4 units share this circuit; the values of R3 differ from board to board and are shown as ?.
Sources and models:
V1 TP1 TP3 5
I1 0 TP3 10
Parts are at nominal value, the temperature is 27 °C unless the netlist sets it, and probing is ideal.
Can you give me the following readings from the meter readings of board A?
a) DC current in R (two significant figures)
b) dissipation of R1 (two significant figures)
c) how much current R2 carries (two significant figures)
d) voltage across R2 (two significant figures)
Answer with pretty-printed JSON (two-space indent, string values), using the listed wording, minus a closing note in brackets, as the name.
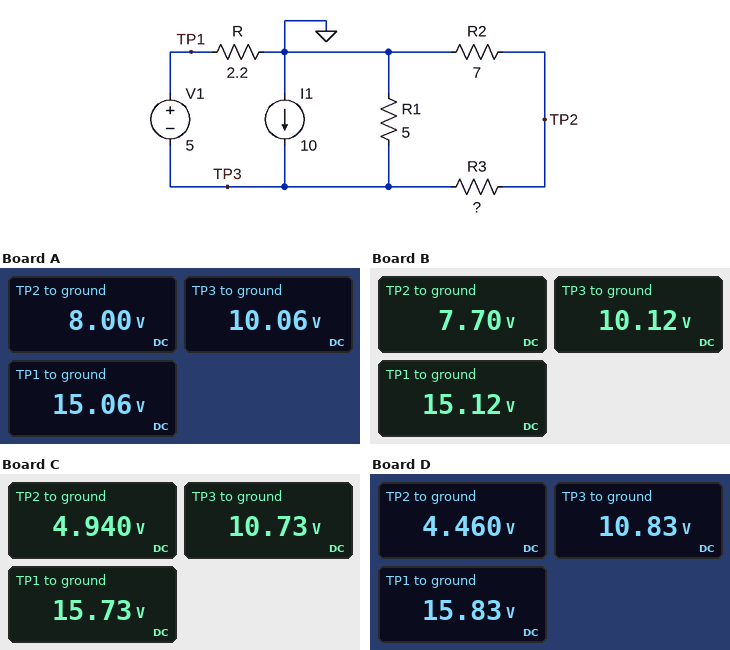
{
  "DC current in R": "6.8 A",
  "dissipation of R1": "20 W",
  "how much current R2 carries": "1.1 A",
  "voltage across R2": "8.0 V"
}
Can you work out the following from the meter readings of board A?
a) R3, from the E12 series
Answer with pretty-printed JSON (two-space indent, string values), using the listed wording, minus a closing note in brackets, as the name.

{
  "R3, from the E12 series": "1.8 Ω"
}
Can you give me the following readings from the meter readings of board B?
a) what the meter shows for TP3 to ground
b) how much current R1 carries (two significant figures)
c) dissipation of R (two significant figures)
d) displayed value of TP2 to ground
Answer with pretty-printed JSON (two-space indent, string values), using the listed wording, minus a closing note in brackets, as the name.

{
  "what the meter shows for TP3 to ground": "10.12 V",
  "how much current R1 carries": "2.0 A",
  "dissipation of R": "100 W",
  "displayed value of TP2 to ground": "7.70 V"
}
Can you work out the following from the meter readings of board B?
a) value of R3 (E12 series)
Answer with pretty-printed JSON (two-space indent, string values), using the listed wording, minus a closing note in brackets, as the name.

{
  "value of R3": "2.2 Ω"
}
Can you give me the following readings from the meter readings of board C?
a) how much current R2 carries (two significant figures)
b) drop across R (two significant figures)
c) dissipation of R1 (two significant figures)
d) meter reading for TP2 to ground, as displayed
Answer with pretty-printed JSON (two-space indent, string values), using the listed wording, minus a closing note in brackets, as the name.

{
  "how much current R2 carries": "710 mA",
  "drop across R": "16 V",
  "dissipation of R1": "23 W",
  "meter reading for TP2 to ground, as displayed": "4.940 V"
}
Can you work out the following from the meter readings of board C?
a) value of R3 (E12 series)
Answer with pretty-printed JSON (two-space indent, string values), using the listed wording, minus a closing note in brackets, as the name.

{
  "value of R3": "8.2 Ω"
}
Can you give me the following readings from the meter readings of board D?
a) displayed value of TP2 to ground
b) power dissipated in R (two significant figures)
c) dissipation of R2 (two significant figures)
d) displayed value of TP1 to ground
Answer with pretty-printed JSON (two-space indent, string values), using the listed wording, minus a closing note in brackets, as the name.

{
  "displayed value of TP2 to ground": "4.460 V",
  "power dissipated in R": "110 W",
  "dissipation of R2": "2.8 W",
  "displayed value of TP1 to ground": "15.83 V"
}
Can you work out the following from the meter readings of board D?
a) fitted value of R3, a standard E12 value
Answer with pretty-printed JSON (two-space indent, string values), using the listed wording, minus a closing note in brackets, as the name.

{
  "fitted value of R3, a standard E12 value": "10 Ω"
}
